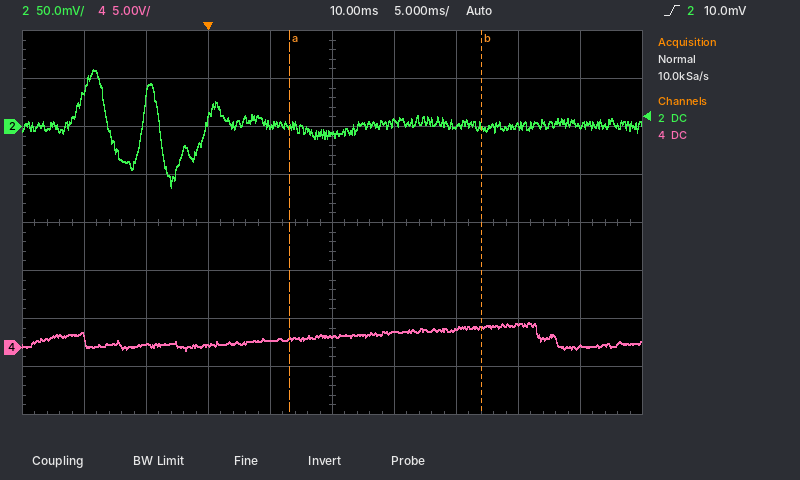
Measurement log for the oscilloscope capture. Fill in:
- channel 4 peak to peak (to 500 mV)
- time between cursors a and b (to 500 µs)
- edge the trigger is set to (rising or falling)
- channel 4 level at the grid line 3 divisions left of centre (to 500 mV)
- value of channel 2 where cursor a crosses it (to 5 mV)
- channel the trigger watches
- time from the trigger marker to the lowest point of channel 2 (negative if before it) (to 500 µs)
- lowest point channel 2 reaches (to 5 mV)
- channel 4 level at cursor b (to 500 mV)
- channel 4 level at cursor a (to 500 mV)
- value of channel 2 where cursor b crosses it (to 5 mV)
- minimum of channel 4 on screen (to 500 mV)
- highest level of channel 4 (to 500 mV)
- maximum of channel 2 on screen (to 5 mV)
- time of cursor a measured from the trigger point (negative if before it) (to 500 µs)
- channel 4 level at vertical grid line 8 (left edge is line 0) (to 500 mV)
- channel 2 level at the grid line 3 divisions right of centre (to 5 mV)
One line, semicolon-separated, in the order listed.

3.0 V; 15.5 ms; rising; 500 mV; 0 mV; channel 2; -3.0 ms; -65 mV; 2.0 V; 1.0 V; 0 mV; -500 mV; 2.5 V; 60 mV; +6.5 ms; 2.5 V; 0 mV
